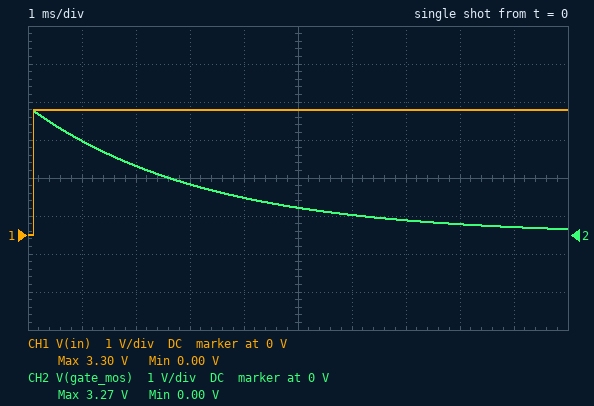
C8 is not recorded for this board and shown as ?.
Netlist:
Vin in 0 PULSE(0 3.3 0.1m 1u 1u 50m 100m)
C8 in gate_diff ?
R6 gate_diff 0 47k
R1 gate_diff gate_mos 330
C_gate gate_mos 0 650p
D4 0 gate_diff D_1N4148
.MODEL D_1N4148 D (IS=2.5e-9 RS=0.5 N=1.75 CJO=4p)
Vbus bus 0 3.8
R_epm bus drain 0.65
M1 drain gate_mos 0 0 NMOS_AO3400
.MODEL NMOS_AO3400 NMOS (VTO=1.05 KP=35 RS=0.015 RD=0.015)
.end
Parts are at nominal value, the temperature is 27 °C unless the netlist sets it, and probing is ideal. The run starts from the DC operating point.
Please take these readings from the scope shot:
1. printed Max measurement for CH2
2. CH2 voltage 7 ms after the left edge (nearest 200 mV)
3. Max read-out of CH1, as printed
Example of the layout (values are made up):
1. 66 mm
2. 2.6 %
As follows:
1. 3.27 V
2. 400 mV
3. 3.30 V
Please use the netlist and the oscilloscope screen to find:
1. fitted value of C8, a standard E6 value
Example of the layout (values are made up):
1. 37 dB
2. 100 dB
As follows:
1. 68 nF
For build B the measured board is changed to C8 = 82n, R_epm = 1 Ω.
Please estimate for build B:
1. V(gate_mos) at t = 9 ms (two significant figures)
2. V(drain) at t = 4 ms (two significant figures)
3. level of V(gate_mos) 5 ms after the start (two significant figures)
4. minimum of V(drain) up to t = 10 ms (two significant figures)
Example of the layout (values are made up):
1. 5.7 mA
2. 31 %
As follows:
1. 330 mV
2. 3.4 V
3. 930 mV
4. 160 mV
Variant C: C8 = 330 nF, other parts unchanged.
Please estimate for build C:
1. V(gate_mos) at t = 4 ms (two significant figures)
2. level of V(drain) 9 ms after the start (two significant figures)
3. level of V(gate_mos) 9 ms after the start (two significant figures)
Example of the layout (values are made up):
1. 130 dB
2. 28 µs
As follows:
1. 2.6 V
2. 400 mV
3. 1.9 V
